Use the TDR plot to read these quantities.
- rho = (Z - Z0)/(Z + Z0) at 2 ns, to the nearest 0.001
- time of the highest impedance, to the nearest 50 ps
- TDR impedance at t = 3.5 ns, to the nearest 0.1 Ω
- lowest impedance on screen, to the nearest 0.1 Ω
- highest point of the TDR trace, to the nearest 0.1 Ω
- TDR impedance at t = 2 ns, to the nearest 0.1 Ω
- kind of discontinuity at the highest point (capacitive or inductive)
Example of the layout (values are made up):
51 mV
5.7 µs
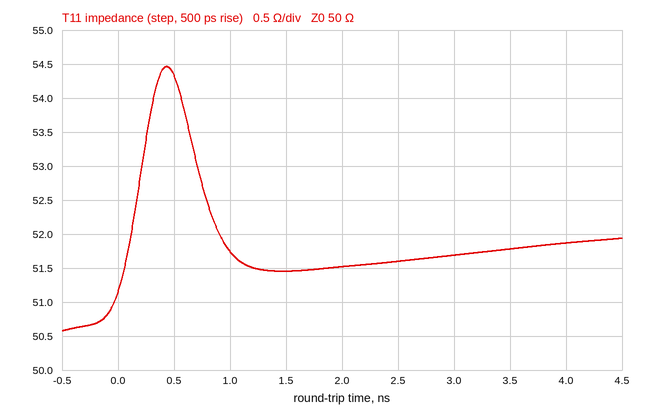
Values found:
+0.015
450 ps
51.8 Ω
50.6 Ω
54.5 Ω
51.5 Ω
inductive
